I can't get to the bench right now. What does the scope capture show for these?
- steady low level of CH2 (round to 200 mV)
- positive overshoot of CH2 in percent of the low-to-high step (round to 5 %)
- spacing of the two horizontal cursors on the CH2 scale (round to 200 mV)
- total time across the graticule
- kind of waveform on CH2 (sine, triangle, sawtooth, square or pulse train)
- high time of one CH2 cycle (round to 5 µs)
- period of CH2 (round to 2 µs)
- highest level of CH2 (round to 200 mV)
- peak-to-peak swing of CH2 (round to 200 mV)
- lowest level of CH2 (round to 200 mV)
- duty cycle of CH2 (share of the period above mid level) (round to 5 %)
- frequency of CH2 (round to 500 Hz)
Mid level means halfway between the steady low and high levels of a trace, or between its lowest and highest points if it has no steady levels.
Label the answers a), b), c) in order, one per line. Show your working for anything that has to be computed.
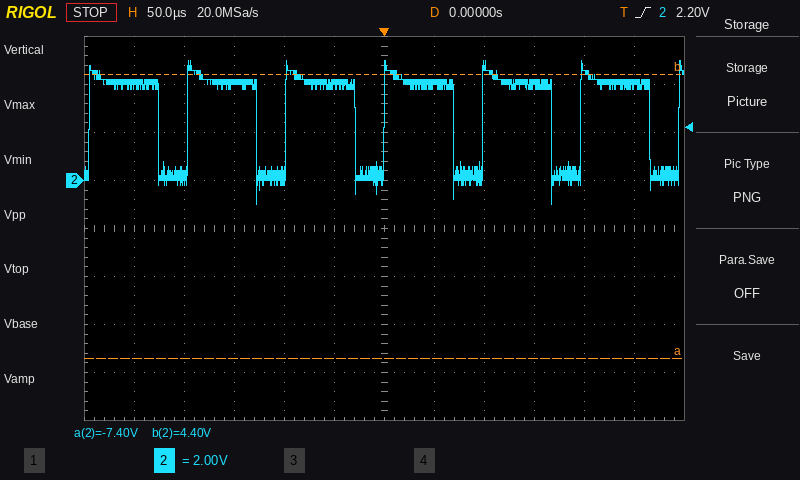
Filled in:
a) 200 mV
b) 25 %
c) 11.8 V
d) 600 µs
e) pulse train
f) 70 µs
g) 98 µs
h) 5.0 V
i) 5.0 V − (-1.0 V) = 6.0 V
j) -1.0 V
k) 70 µs / 98 µs ≈ 71.4 %, so 70 % to the nearest 5 %
l) 1 / 98 µs ≈ 10.2 kHz, so 10.0 kHz to the nearest 500 Hz
